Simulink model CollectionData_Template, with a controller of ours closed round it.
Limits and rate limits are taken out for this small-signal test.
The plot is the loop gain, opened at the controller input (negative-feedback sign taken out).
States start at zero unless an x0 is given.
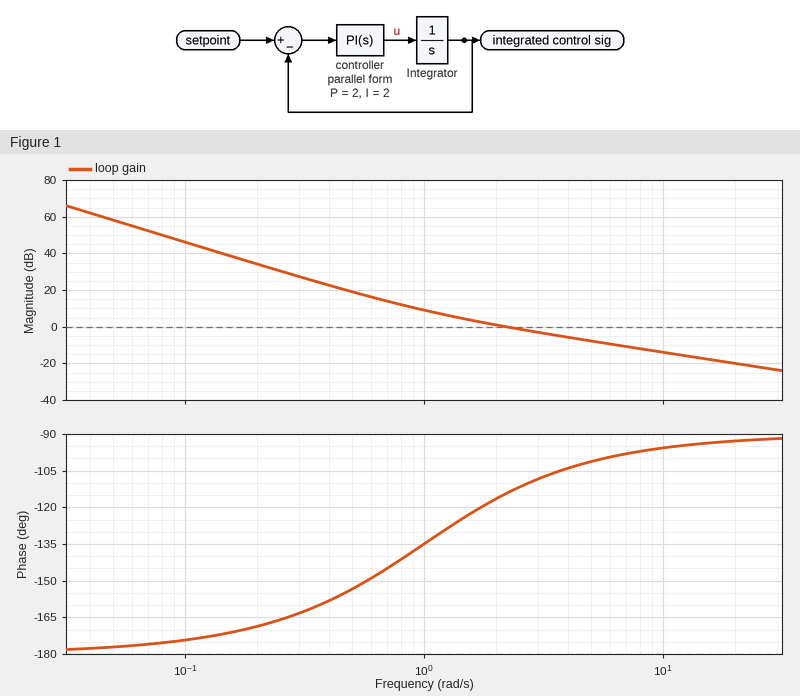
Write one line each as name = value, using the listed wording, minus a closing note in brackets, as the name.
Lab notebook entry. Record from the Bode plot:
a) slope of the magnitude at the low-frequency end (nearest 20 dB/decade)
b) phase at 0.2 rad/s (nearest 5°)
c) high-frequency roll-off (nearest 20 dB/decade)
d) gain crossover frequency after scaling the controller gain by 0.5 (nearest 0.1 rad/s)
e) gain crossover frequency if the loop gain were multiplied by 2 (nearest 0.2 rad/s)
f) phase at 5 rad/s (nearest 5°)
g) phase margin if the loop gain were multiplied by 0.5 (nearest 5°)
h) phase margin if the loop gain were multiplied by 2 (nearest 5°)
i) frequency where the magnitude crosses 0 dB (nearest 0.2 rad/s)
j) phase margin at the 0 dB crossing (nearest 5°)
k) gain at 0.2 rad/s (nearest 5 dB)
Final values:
slope of the magnitude at the low-frequency end = -40 dB/decade
phase at 0.2 rad/s = -170°
high-frequency roll-off = -20 dB/decade
gain crossover frequency after scaling the controller gain by 0.5 = 1.3 rad/s
gain crossover frequency if the loop gain were multiplied by 2 = 4.2 rad/s
phase at 5 rad/s = -100°
phase margin if the loop gain were multiplied by 0.5 = 50°
phase margin if the loop gain were multiplied by 2 = 75°
frequency where the magnitude crosses 0 dB = 2.2 rad/s
phase margin at the 0 dB crossing = 65°
gain at 0.2 rad/s = 35 dB
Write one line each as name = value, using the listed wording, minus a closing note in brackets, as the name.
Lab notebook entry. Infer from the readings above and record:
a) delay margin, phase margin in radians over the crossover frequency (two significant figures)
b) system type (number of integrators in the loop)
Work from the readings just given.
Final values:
delay margin, phase margin in radians over the crossover frequency = 0.52 s
system type = 2
